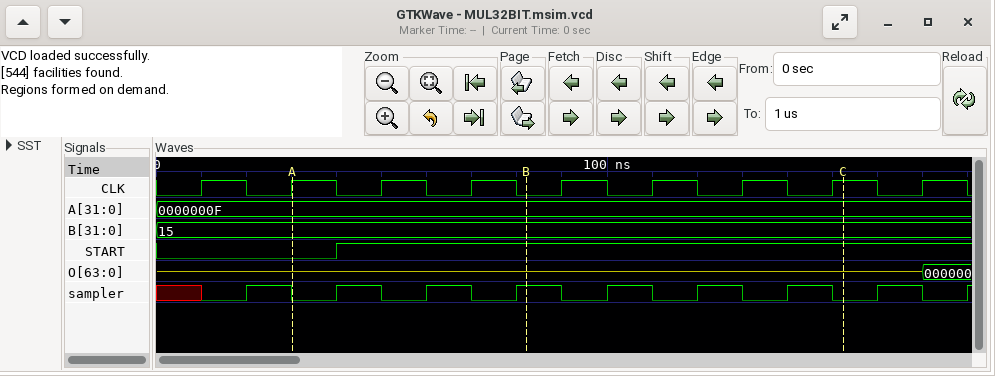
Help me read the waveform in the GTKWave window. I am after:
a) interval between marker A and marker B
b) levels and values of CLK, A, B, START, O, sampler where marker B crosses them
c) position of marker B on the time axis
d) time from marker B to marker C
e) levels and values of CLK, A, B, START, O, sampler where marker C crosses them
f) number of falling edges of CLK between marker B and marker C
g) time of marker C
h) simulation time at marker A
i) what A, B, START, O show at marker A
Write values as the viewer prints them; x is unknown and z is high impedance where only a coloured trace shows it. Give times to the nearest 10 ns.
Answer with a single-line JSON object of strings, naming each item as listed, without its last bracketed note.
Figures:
{"interval between marker A and marker B": "50 ns", "levels and values of CLK, A, B, START, O, sampler where marker B crosses them": "CLK=0, A=0000000F, B=15, START=1, O=z, sampler=1", "position of marker B on the time axis": "80 ns", "time from marker B to marker C": "70 ns", "levels and values of CLK, A, B, START, O, sampler where marker C crosses them": "CLK=1, A=0000000F, B=15, START=1, O=z, sampler=0", "number of falling edges of CLK between marker B and marker C": "3", "time of marker C": "150 ns", "simulation time at marker A": "30 ns", "what A, B, START, O show at marker A": "A=0000000F, B=15, START=0, O=z"}
